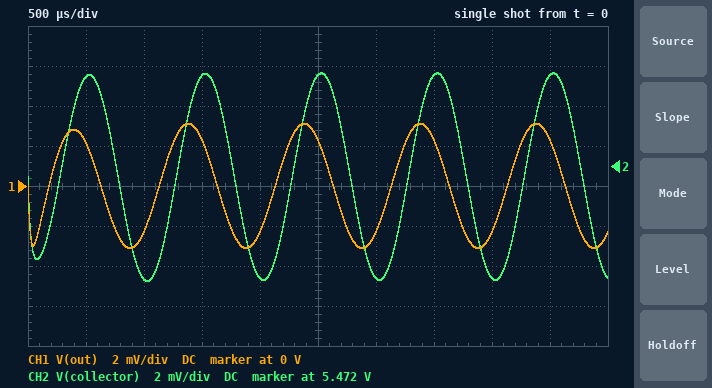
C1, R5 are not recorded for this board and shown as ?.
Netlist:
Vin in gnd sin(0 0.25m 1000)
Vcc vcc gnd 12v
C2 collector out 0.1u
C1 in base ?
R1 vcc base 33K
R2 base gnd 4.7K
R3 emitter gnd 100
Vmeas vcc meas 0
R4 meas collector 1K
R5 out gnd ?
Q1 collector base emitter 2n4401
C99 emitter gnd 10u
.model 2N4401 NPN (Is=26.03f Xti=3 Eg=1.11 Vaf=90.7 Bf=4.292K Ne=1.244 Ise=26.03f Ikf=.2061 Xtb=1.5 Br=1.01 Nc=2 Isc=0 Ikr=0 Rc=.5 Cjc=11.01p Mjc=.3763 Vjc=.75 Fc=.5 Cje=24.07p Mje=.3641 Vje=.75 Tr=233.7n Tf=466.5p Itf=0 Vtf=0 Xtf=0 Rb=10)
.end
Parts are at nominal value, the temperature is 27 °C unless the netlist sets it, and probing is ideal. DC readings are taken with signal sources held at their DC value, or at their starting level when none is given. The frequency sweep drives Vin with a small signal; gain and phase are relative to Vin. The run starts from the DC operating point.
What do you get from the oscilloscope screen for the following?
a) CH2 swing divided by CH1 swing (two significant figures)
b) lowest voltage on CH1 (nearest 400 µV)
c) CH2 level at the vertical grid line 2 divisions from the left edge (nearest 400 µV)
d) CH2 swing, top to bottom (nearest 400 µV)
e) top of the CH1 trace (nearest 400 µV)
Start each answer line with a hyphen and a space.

- 1.7
- -3.2 mV
- 5.4664 V
- 10.4 mV
- 3.2 mV
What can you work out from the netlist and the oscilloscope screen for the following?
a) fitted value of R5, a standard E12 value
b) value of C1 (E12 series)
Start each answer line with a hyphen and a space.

- 1.2 kΩ
- 56 nF
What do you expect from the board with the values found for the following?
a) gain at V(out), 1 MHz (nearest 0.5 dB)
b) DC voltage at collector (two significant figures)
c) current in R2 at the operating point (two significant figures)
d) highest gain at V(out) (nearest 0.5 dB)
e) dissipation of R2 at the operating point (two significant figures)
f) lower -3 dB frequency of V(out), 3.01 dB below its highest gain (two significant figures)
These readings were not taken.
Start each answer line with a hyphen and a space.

- 42.0 dB
- 5.5 V
- 280 µA
- 42.0 dB
- 380 µW
- 7.6 kHz
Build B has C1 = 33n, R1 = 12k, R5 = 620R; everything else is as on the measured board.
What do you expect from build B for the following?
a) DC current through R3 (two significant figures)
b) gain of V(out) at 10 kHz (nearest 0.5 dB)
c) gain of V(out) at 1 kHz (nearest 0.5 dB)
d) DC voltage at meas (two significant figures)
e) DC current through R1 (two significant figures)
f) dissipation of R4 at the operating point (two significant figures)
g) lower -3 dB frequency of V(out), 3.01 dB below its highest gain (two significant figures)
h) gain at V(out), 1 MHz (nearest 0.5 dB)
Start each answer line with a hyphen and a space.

- 11 mA
- -18.5 dB
- -47.0 dB
- 12 V
- 850 µA
- 120 mW
- 190 kHz
- 7.5 dB
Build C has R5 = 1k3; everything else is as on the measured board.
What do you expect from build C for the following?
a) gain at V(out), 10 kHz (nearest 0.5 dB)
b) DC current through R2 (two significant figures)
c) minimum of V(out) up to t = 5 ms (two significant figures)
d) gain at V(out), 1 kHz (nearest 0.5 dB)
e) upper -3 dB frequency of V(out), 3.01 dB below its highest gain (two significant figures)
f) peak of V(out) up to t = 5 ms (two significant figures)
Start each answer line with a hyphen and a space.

- 40.5 dB
- 280 µA
- -3.3 mV
- 22.5 dB
- 14 MHz
- 3.3 mV
